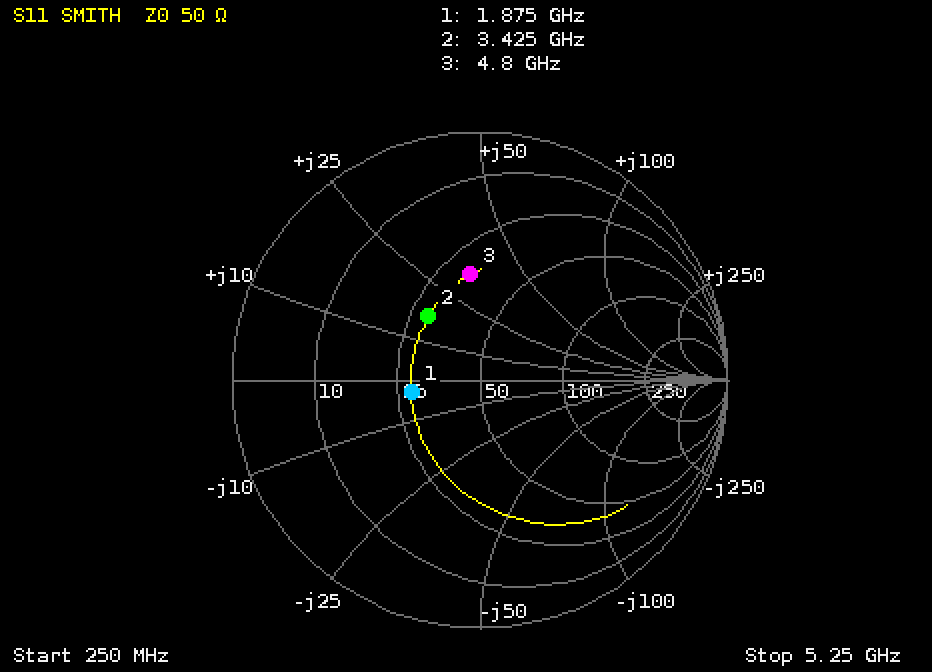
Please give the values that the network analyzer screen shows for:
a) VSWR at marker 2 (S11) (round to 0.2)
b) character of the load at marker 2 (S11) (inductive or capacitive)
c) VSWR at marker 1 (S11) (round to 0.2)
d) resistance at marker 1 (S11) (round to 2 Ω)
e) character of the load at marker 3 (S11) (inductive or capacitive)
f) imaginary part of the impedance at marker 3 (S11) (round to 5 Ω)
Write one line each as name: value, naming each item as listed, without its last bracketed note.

VSWR at marker 2 (S11): 2.0
character of the load at marker 2 (S11): inductive
VSWR at marker 1 (S11): 1.8
resistance at marker 1 (S11): 28 Ω
character of the load at marker 3 (S11): inductive
imaginary part of the impedance at marker 3 (S11): +35 Ω
